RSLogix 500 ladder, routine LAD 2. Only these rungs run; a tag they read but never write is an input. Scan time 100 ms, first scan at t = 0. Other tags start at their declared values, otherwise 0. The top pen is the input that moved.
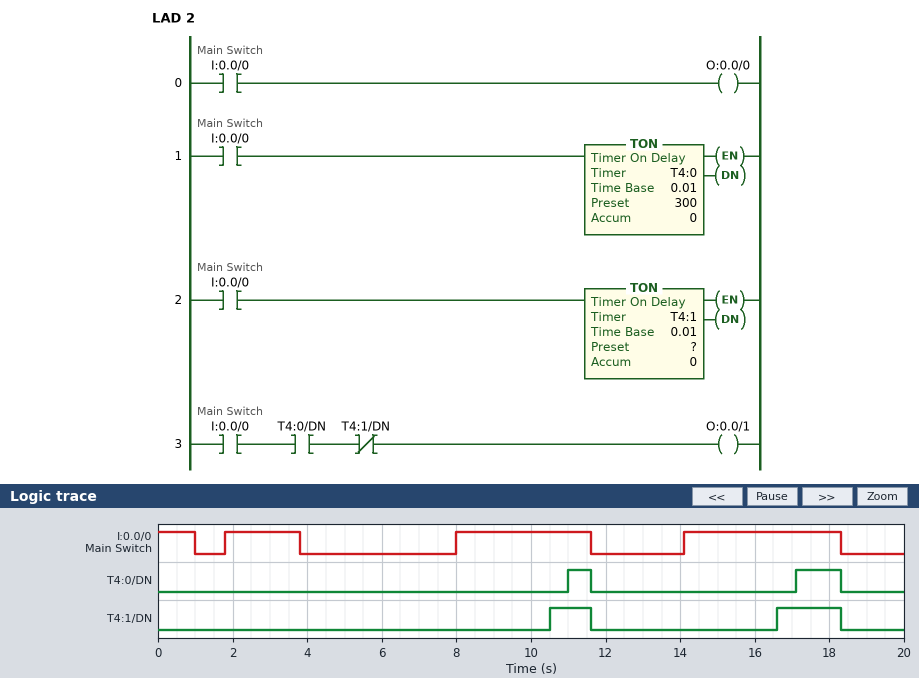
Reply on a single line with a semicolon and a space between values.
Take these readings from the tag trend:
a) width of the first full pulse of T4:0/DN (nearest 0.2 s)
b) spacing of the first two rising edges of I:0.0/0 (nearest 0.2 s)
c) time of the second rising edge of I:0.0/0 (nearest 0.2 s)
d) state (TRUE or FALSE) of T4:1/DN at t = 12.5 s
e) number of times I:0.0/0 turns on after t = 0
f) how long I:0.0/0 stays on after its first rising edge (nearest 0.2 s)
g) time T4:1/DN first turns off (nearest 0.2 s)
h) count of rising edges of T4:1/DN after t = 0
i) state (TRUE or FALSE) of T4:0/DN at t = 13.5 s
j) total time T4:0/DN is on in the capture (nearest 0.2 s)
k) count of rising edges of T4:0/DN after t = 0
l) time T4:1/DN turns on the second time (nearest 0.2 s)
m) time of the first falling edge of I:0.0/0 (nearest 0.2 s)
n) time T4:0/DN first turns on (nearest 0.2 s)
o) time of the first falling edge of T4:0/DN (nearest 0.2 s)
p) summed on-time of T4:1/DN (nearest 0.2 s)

0.6 s; 6.2 s; 8.0 s; FALSE; 3; 2.0 s; 11.6 s; 2; FALSE; 1.8 s; 2; 16.6 s; 1.0 s; 11.0 s; 11.6 s; 2.8 s
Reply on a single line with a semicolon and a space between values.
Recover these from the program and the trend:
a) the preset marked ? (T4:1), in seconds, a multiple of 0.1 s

2.5 s
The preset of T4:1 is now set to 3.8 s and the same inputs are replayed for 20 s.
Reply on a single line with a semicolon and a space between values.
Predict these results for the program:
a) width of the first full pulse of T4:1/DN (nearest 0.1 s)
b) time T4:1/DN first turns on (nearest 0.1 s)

0.4 s; 17.9 s
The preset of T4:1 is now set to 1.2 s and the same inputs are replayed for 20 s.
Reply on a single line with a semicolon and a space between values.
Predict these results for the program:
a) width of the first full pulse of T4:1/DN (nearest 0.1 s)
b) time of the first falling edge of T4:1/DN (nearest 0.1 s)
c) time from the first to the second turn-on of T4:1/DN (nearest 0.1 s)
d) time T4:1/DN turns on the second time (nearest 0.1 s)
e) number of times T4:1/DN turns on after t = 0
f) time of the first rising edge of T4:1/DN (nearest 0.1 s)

0.8 s; 3.8 s; 6.2 s; 9.2 s; 3; 3.0 s
